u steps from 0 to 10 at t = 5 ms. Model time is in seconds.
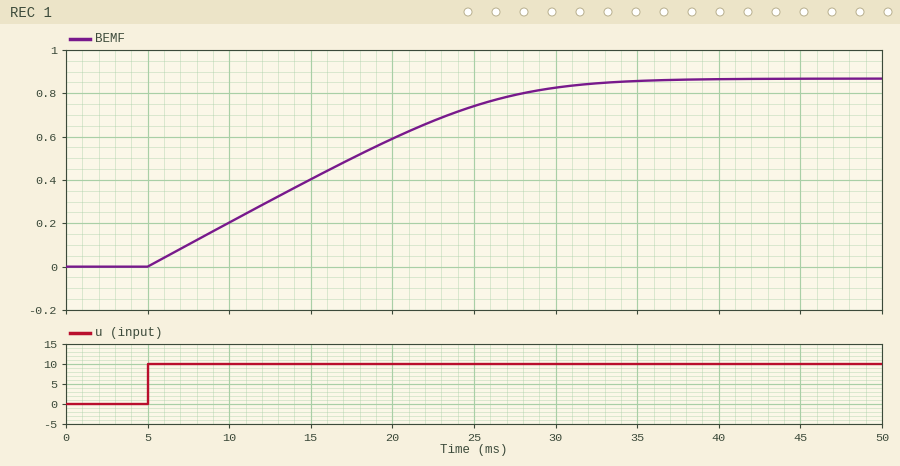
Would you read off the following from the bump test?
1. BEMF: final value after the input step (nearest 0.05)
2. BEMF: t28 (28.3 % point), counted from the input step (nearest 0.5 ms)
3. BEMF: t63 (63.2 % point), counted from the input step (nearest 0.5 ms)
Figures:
0.85
6.0 ms
14.0 ms
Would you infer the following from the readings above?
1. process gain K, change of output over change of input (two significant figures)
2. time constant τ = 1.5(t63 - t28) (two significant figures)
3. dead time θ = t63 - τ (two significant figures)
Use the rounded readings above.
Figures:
0.085
12 ms
2.0 ms
